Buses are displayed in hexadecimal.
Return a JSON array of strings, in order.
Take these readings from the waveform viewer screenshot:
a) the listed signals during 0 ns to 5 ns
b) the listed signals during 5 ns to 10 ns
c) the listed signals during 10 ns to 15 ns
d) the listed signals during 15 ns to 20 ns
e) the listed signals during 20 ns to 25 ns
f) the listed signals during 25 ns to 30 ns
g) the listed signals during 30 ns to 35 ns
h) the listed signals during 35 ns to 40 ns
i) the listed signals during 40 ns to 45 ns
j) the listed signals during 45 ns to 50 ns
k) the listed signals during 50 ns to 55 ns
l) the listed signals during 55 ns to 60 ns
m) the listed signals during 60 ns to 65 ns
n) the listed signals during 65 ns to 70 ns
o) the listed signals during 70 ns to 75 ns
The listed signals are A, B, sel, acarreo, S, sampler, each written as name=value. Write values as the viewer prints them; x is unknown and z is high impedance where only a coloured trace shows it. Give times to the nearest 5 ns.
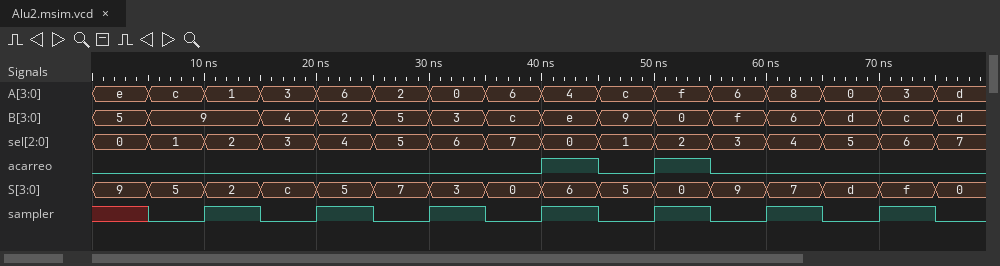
["A=e, B=5, sel=0, acarreo=0, S=9, sampler=x", "A=c, B=9, sel=1, acarreo=0, S=5, sampler=0", "A=1, B=9, sel=2, acarreo=0, S=2, sampler=1", "A=3, B=4, sel=3, acarreo=0, S=c, sampler=0", "A=6, B=2, sel=4, acarreo=0, S=5, sampler=1", "A=2, B=5, sel=5, acarreo=0, S=7, sampler=0", "A=0, B=3, sel=6, acarreo=0, S=3, sampler=1", "A=6, B=c, sel=7, acarreo=0, S=0, sampler=0", "A=4, B=e, sel=0, acarreo=1, S=6, sampler=1", "A=c, B=9, sel=1, acarreo=0, S=5, sampler=0", "A=f, B=0, sel=2, acarreo=1, S=0, sampler=1", "A=6, B=f, sel=3, acarreo=0, S=9, sampler=0", "A=8, B=6, sel=4, acarreo=0, S=7, sampler=1", "A=0, B=d, sel=5, acarreo=0, S=d, sampler=0", "A=3, B=c, sel=6, acarreo=0, S=f, sampler=1"]
